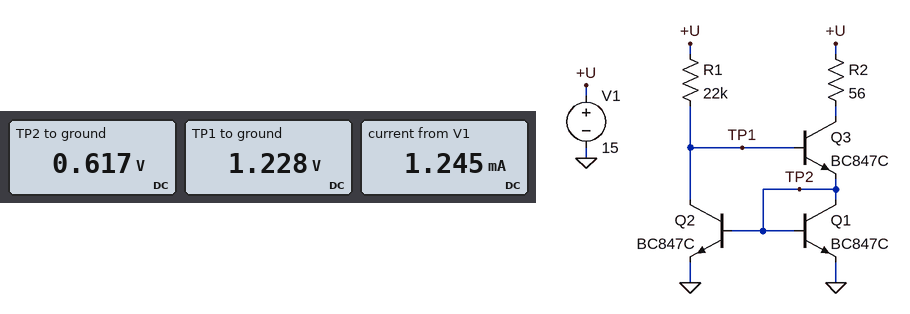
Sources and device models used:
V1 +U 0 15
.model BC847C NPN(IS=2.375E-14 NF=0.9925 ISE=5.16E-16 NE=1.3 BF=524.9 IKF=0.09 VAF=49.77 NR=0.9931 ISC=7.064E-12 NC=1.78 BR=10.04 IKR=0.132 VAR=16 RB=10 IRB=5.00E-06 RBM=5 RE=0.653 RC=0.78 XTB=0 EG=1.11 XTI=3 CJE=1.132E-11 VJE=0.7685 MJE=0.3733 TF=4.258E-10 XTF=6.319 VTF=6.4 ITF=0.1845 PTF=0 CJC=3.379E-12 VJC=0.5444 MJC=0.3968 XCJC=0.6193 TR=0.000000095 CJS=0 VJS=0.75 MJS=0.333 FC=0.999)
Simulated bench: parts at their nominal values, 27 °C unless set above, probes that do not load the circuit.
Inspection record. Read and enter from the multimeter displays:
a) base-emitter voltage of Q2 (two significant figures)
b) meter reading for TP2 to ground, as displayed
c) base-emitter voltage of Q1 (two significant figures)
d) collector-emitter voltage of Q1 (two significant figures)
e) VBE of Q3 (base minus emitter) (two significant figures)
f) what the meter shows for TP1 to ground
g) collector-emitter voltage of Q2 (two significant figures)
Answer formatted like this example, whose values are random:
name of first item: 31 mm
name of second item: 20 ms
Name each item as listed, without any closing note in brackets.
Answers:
base-emitter voltage of Q2: 620 mV
meter reading for TP2 to ground, as displayed: 0.617 V
base-emitter voltage of Q1: 620 mV
collector-emitter voltage of Q1: 620 mV
VBE of Q3 (base minus emitter): 610 mV
what the meter shows for TP1 to ground: 1.228 V
collector-emitter voltage of Q2: 1.2 V
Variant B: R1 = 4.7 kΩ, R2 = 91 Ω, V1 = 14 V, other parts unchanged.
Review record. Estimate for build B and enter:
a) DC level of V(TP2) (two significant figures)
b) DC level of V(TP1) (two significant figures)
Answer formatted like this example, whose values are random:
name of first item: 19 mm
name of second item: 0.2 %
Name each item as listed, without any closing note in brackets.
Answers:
DC level of V(TP2): 660 mV
DC level of V(TP1): 1.3 V
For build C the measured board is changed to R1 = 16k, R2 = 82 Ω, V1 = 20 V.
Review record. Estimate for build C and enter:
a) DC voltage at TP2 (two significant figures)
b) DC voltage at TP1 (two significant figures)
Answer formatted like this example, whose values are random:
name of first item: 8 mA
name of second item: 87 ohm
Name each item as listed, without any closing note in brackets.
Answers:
DC voltage at TP2: 630 mV
DC voltage at TP1: 1.3 V
